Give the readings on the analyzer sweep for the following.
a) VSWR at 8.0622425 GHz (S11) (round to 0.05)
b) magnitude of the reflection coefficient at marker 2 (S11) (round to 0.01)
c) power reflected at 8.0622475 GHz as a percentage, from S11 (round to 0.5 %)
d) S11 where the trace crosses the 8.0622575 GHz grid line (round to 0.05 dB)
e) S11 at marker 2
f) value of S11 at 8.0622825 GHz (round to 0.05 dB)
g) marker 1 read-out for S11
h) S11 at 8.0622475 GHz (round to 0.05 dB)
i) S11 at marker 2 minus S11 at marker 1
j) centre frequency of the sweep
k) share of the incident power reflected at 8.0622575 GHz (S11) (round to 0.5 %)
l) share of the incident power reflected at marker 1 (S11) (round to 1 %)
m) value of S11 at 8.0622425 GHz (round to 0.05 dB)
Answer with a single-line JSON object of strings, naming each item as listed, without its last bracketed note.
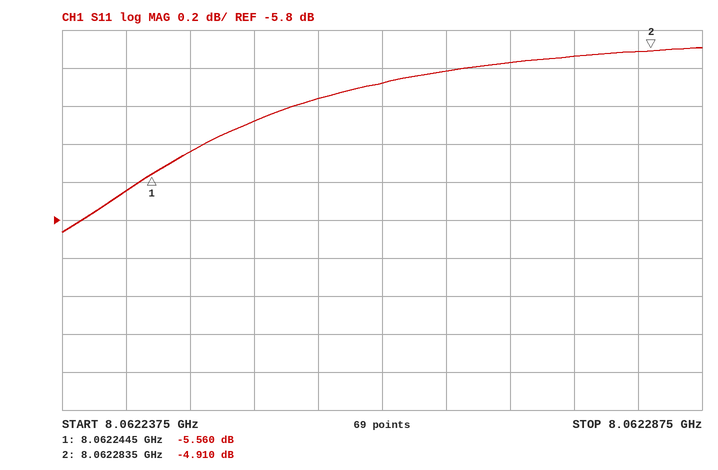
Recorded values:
{"VSWR at 8.0622425 GHz (S11)": "3.20", "magnitude of the reflection coefficient at marker 2 (S11)": "0.57", "power reflected at 8.0622475 GHz as a percentage, from S11": "28.5 %", "S11 where the trace crosses the 8.0622575 GHz grid line": "-5.15 dB", "S11 at marker 2": "-4.910 dB", "value of S11 at 8.0622825 GHz": "-4.90 dB", "marker 1 read-out for S11": "-5.560 dB", "S11 at 8.0622475 GHz": "-5.45 dB", "S11 at marker 2 minus S11 at marker 1": "0.650 dB", "centre frequency of the sweep": "8.0622625 GHz", "share of the incident power reflected at 8.0622575 GHz (S11)": "30.5 %", "share of the incident power reflected at marker 1 (S11)": "28 %", "value of S11 at 8.0622425 GHz": "-5.65 dB"}
